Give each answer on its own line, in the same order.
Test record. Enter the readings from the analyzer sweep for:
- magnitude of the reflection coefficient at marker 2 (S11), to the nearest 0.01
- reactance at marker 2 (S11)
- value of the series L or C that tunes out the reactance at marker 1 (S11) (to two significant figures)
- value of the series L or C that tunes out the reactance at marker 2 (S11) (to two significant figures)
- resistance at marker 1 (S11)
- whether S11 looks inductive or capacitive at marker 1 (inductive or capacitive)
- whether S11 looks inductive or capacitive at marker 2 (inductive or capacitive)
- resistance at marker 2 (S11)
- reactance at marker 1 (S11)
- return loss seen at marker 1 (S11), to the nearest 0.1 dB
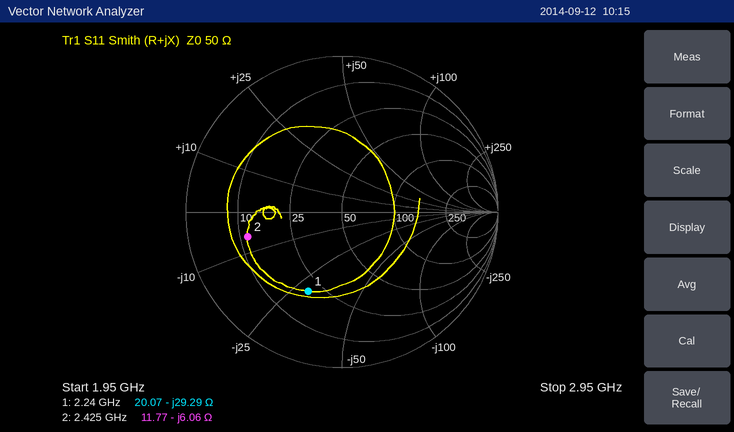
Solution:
0.62
-6.06 Ω
2.1 nH
400 pH
20.07 Ω
capacitive
capacitive
11.77 Ω
-29.29 Ω
5.2 dB
